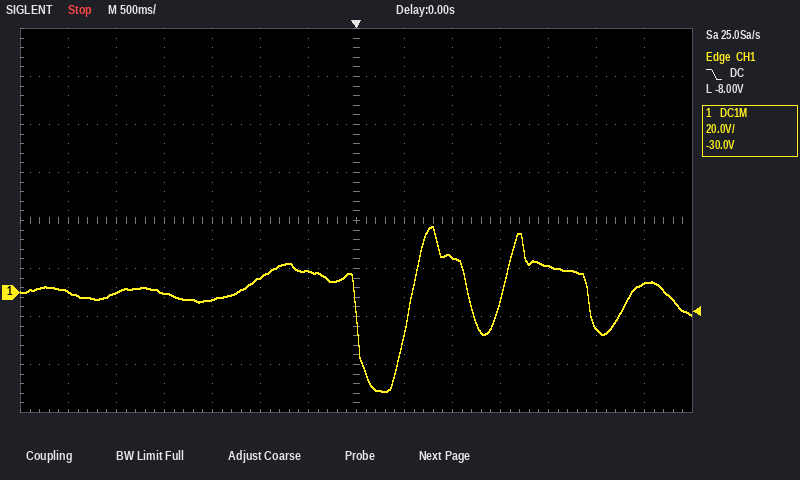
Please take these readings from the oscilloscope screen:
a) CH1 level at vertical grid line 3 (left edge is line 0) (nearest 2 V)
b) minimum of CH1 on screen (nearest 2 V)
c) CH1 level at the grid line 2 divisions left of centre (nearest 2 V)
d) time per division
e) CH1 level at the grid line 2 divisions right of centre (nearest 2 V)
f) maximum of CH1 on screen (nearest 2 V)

0 V
-42 V
6 V
500 ms
14 V
28 V
